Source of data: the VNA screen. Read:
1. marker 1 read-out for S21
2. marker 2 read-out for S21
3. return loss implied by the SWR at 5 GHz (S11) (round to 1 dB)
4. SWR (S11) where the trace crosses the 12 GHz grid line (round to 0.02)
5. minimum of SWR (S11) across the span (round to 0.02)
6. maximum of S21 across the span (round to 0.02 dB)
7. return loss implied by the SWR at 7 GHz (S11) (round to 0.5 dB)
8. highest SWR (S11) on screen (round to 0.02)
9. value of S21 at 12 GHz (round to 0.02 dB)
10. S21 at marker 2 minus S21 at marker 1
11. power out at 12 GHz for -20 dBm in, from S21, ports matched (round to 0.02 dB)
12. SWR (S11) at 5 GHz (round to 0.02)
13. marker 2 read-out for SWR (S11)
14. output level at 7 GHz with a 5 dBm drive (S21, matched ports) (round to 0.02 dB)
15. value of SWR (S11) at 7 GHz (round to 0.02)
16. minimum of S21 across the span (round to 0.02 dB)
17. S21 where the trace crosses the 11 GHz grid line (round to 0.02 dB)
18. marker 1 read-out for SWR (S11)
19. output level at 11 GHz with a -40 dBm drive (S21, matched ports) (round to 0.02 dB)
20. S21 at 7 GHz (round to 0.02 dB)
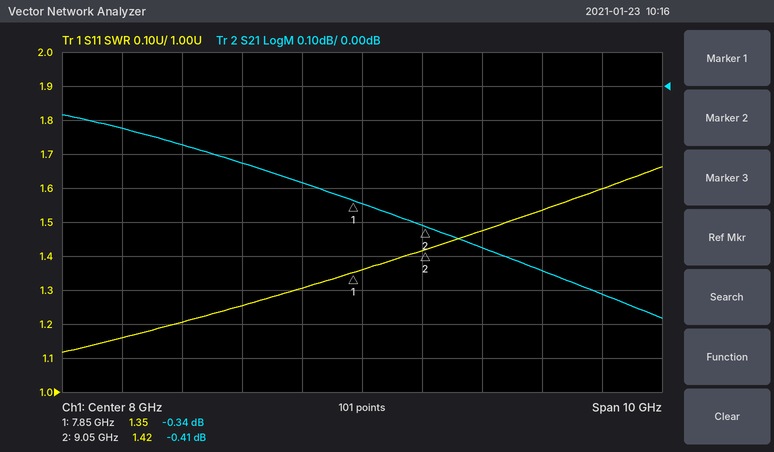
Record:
-0.34 dB
-0.41 dB
21 dB
1.60
1.12
-0.08 dB
17.5 dB
1.66
-0.62 dB
-0.07 dB
-20.62 dBm
1.20
1.42
4.72 dBm
1.30
-0.68 dB
-0.54 dB
1.35
-40.54 dBm
-0.28 dB
